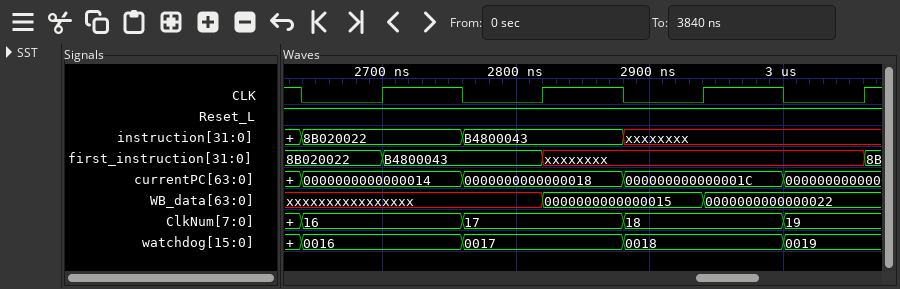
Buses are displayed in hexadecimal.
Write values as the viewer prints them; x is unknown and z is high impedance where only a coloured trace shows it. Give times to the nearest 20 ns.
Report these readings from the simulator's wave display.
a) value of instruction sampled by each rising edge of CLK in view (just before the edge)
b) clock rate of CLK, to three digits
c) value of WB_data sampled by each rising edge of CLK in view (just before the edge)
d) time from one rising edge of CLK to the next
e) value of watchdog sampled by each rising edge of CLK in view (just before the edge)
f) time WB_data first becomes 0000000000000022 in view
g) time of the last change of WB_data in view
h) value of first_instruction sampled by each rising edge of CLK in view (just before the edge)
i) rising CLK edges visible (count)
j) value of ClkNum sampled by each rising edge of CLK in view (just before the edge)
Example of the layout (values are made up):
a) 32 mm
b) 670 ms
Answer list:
a) 8B020022, B4800043, xxxxxxxx, xxxxxxxx
b) 8.33 MHz
c) xxxxxxxxxxxxxxxx, xxxxxxxxxxxxxxxx, 0000000000000015, 0000000000000022
d) 120 ns
e) 0016, 0017, 0018, 0019
f) 2940 ns
g) 2940 ns
h) 8B020022, B4800043, xxxxxxxx, xxxxxxxx
i) 4
j) 16, 17, 18, 19
